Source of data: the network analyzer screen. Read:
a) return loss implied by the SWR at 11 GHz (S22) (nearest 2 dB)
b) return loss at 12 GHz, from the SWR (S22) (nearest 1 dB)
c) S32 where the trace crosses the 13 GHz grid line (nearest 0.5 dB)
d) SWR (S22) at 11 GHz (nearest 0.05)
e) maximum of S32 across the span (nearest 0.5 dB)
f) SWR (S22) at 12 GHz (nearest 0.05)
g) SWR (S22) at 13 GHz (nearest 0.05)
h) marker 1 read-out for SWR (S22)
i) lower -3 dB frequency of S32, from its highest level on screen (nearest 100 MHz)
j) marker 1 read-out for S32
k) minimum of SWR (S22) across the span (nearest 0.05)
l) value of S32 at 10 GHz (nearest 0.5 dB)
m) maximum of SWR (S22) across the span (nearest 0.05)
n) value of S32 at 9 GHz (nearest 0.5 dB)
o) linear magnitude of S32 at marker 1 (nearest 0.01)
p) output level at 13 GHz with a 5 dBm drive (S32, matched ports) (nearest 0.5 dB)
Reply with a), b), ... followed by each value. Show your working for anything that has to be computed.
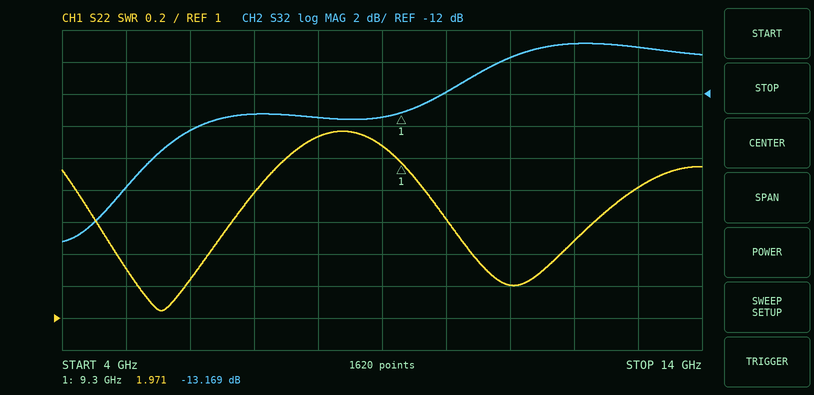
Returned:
a) −20 log10((1.2 − 1)/(1.2 + 1)) ≈ 20.8 dB, so 20 dB to the nearest 2 dB
b) −20 log10((1.5 − 1)/(1.5 + 1)) ≈ 14 dB
c) -9.0 dB
d) 1.20
e) -9.0 dB
f) 1.50
g) 1.80
h) 1.971
i) 10.0 GHz
j) -13.169 dB
k) 1.05
l) -12.0 dB
m) 2.15
n) -13.5 dB
o) 10^(-13.169/20) ≈ 0.22
p) 5 dBm + (-9.0 dB) = -4.0 dBm
